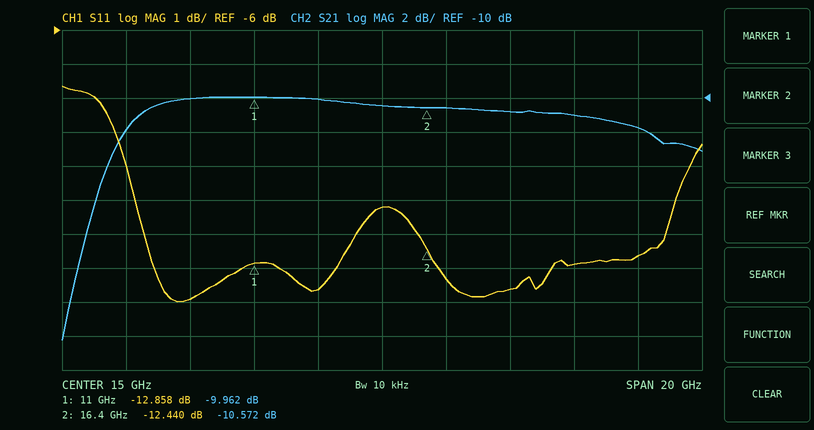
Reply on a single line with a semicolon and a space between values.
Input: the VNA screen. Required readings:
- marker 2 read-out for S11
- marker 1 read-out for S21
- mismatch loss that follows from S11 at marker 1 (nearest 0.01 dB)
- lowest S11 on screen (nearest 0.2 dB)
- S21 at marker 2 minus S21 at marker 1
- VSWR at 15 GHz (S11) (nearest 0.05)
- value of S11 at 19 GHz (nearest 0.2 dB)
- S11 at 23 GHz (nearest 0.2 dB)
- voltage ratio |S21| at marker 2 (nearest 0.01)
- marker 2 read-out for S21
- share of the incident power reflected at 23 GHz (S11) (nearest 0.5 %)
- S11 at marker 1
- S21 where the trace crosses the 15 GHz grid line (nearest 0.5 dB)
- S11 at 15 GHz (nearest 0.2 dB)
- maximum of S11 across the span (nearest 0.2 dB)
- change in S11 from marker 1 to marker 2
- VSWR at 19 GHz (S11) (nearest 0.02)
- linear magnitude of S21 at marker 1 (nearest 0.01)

-12.440 dB; -9.962 dB; 0.23 dB; -14.0 dB; -0.610 dB; 1.75; -13.6 dB; -12.6 dB; 0.30; -10.572 dB; 5.5 %; -12.858 dB; -10.5 dB; -11.2 dB; -7.6 dB; 0.418 dB; 1.52; 0.32
